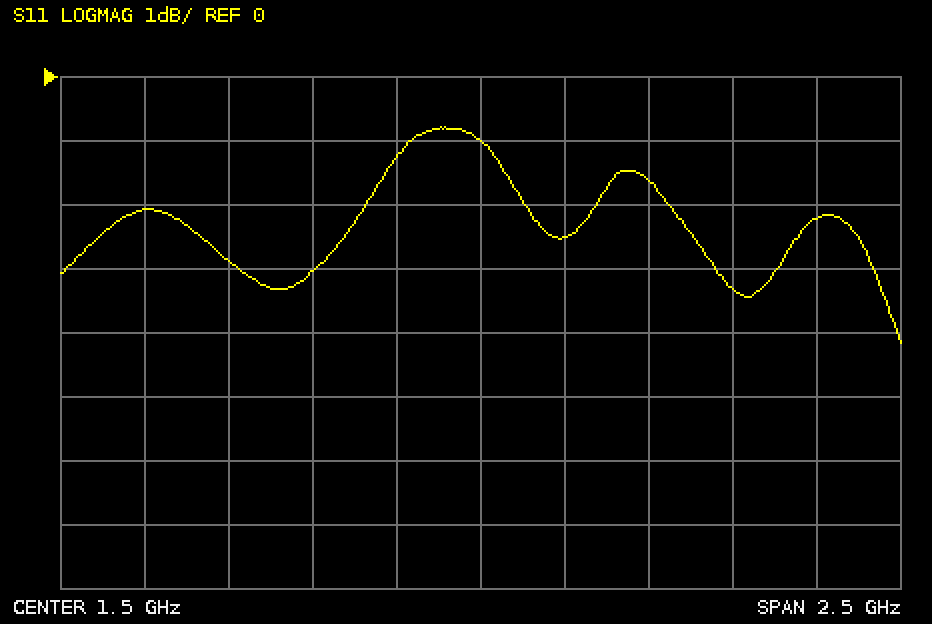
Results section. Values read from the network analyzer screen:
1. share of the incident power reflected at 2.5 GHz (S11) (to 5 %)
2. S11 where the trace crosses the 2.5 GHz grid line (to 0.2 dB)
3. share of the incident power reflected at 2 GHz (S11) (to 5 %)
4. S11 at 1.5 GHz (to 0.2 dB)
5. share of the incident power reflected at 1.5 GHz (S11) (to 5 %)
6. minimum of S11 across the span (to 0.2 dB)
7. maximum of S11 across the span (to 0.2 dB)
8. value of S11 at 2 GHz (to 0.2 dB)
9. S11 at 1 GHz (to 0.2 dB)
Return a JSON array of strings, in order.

["60 %", "-2.2 dB", "70 %", "-1.0 dB", "80 %", "-4.2 dB", "-0.8 dB", "-1.6 dB", "-3.0 dB"]
